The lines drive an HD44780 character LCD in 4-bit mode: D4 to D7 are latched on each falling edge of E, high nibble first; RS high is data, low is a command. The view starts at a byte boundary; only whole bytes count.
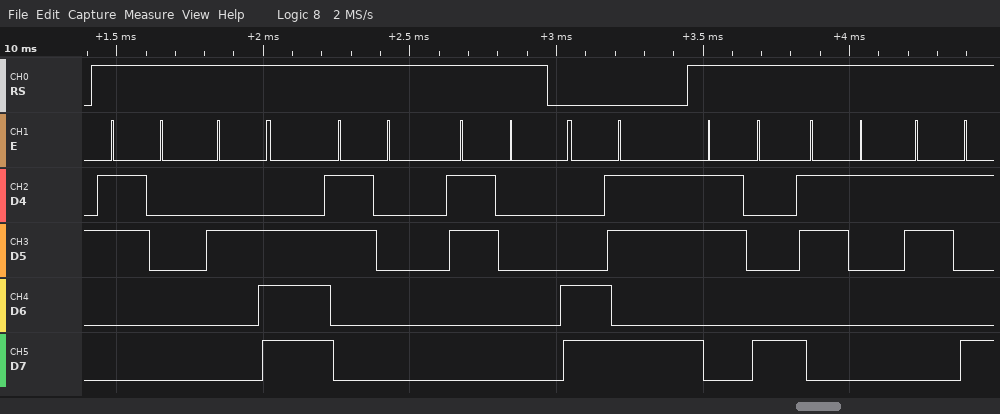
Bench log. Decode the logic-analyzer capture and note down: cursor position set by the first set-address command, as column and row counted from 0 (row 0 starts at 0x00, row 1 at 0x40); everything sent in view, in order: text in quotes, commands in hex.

column 11, row 1
"0.00" 0xCB "819"
